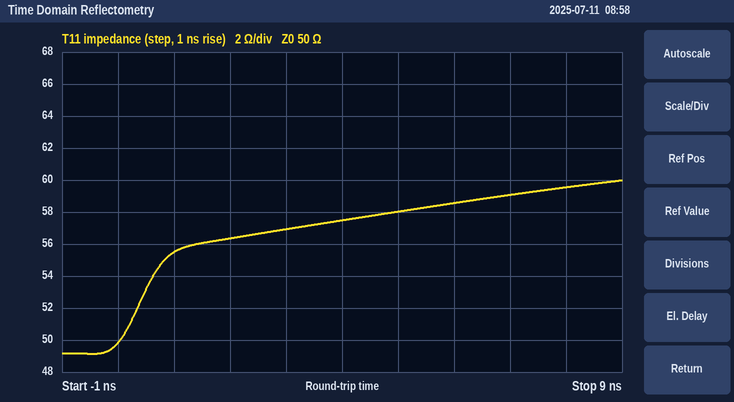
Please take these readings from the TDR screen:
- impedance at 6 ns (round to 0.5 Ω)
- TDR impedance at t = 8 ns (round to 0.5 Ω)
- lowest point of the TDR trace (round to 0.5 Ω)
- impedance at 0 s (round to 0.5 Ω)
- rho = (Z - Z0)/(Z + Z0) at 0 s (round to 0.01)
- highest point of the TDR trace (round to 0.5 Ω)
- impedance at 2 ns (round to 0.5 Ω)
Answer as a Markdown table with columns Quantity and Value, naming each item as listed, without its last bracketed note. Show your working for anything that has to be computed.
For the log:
| Quantity | Value |
|---|---|
| impedance at 6 ns | 58.5 Ω |
| TDR impedance at t = 8 ns | 59.5 Ω |
| lowest point of the TDR trace | 49.0 Ω |
| impedance at 0 s | 50.0 Ω |
| rho = (Z - Z0)/(Z + Z0) at 0 s | (50 − 50)/(50 + 50) ≈ 0.00 |
| highest point of the TDR trace | 60.0 Ω |
| impedance at 2 ns | 56.5 Ω |
